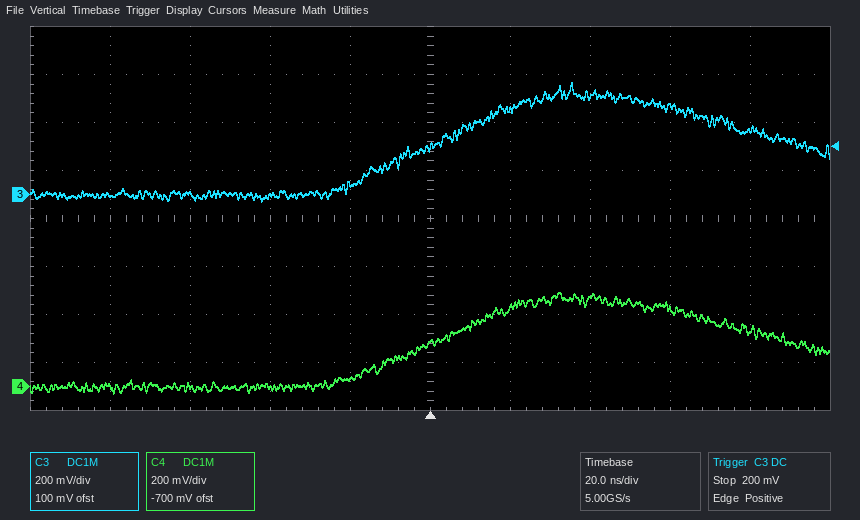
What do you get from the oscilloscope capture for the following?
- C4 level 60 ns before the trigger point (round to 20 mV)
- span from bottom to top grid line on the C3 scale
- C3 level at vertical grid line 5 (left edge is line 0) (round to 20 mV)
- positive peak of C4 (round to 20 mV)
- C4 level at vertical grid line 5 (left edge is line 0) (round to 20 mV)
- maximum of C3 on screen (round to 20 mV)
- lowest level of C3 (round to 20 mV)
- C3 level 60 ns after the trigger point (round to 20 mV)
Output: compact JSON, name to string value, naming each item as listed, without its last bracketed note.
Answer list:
{"C4 level 60 ns before the trigger point": "0 mV", "span from bottom to top grid line on the C3 scale": "1.6 V", "C3 level at vertical grid line 5 (left edge is line 0)": "200 mV", "positive peak of C4": "400 mV", "C4 level at vertical grid line 5 (left edge is line 0)": "180 mV", "maximum of C3 on screen": "460 mV", "lowest level of C3": "-20 mV", "C3 level 60 ns after the trigger point": "360 mV"}
